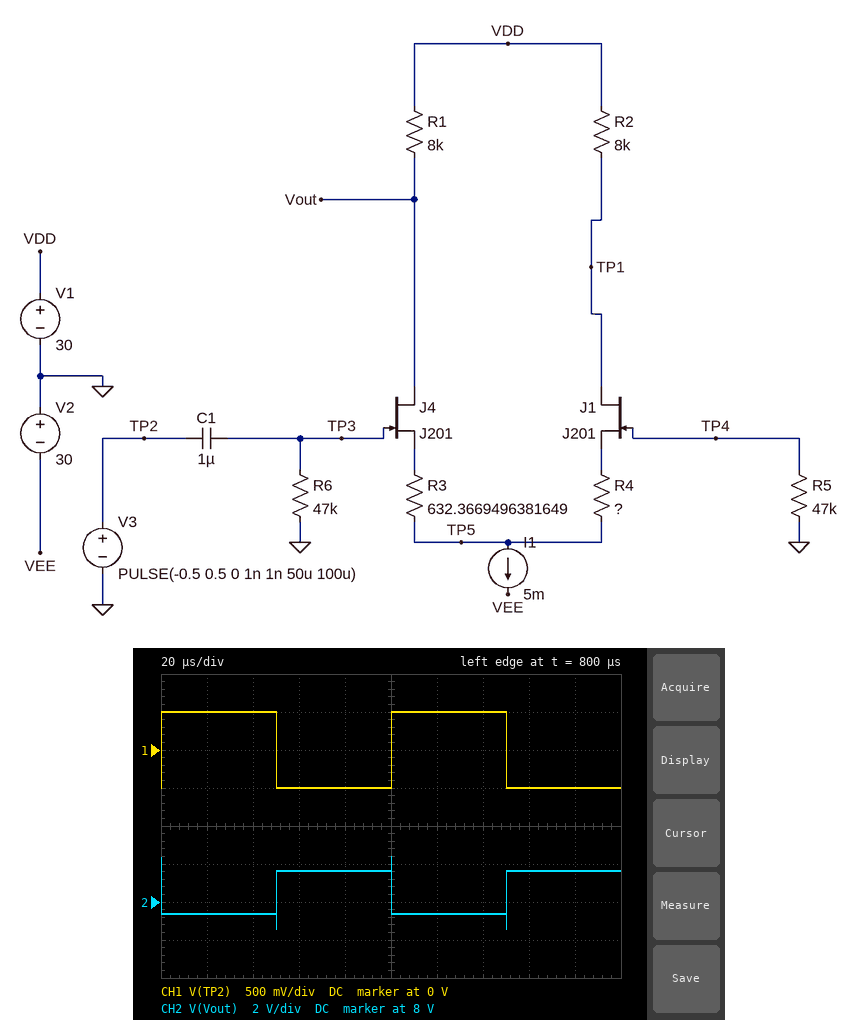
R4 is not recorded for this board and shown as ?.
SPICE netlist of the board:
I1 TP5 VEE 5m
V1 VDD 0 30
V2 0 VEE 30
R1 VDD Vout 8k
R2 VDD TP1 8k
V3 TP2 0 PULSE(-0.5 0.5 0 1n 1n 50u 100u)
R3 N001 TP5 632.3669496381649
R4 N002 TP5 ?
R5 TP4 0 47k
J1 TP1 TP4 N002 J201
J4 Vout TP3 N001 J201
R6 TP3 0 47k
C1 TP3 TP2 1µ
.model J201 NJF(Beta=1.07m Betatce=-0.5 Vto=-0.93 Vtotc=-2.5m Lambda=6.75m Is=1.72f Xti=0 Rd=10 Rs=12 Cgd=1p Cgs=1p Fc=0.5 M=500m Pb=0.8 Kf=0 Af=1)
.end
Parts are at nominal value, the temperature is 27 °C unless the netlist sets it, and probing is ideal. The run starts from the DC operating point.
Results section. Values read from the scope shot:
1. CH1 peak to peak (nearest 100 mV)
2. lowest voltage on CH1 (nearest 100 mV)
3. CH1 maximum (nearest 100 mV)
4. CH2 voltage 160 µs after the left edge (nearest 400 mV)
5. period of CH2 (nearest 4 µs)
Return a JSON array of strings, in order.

["1.0 V", "-500 mV", "500 mV", "9.6 V", "100 µs"]
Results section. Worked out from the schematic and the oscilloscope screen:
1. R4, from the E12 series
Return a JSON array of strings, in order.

["820 Ω"]
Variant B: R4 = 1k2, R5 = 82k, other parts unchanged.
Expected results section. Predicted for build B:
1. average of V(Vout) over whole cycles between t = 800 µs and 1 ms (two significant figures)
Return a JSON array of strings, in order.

["8.0 V"]
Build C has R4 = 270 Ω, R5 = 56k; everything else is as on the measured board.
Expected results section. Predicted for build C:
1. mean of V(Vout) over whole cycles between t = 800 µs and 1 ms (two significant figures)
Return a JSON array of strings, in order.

["10 V"]
